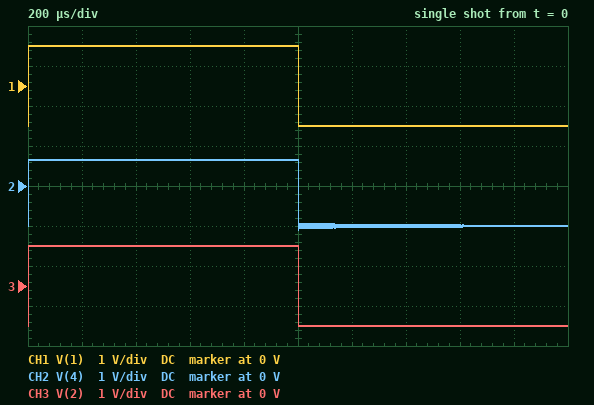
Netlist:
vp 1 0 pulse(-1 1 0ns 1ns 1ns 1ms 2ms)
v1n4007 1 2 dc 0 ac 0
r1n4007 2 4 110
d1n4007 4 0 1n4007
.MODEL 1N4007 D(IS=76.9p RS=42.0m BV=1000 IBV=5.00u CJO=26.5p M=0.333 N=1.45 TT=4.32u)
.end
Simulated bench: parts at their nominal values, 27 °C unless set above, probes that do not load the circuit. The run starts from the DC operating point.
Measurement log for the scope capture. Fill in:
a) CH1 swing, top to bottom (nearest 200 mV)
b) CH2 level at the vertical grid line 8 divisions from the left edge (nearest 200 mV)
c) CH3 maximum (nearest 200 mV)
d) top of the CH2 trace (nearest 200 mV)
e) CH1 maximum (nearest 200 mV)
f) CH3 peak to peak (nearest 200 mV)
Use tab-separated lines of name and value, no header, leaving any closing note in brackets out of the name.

CH1 swing, top to bottom	2.0 V
CH2 level at the vertical grid line 8 divisions from the left edge	-1.0 V
CH3 maximum	1.0 V
top of the CH2 trace	600 mV
CH1 maximum	1.0 V
CH3 peak to peak	2.0 V
